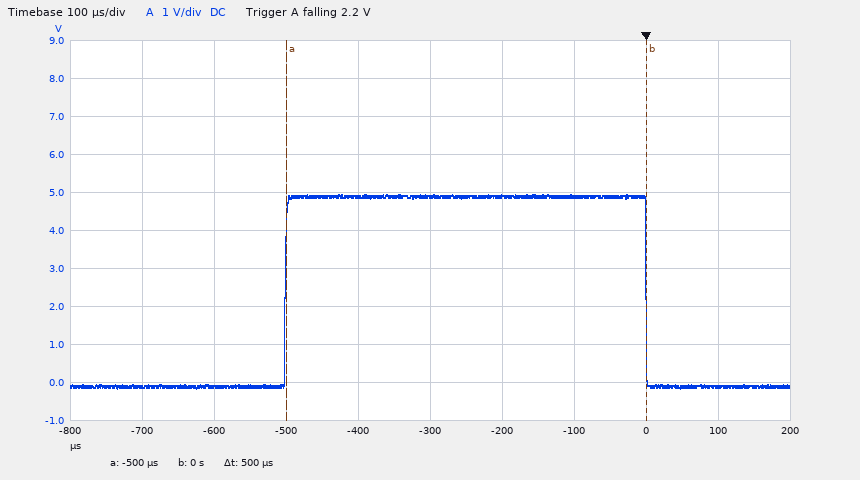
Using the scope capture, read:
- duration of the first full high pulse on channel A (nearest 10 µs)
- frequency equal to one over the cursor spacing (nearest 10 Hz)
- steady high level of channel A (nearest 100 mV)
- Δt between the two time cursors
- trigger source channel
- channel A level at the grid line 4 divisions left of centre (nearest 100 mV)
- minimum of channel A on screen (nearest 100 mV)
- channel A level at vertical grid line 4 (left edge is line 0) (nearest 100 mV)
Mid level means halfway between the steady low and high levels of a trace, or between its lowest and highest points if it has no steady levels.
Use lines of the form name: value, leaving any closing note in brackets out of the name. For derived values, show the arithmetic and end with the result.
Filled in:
duration of the first full high pulse on channel A: 500 µs
frequency equal to one over the cursor spacing: 1 / 500 µs ≈ 2.00 kHz
steady high level of channel A: 4.9 V
Δt between the two time cursors: 500 µs
trigger source channel: channel A
channel A level at the grid line 4 divisions left of centre: -100 mV
minimum of channel A on screen: -200 mV
channel A level at vertical grid line 4 (left edge is line 0): 4.9 V
